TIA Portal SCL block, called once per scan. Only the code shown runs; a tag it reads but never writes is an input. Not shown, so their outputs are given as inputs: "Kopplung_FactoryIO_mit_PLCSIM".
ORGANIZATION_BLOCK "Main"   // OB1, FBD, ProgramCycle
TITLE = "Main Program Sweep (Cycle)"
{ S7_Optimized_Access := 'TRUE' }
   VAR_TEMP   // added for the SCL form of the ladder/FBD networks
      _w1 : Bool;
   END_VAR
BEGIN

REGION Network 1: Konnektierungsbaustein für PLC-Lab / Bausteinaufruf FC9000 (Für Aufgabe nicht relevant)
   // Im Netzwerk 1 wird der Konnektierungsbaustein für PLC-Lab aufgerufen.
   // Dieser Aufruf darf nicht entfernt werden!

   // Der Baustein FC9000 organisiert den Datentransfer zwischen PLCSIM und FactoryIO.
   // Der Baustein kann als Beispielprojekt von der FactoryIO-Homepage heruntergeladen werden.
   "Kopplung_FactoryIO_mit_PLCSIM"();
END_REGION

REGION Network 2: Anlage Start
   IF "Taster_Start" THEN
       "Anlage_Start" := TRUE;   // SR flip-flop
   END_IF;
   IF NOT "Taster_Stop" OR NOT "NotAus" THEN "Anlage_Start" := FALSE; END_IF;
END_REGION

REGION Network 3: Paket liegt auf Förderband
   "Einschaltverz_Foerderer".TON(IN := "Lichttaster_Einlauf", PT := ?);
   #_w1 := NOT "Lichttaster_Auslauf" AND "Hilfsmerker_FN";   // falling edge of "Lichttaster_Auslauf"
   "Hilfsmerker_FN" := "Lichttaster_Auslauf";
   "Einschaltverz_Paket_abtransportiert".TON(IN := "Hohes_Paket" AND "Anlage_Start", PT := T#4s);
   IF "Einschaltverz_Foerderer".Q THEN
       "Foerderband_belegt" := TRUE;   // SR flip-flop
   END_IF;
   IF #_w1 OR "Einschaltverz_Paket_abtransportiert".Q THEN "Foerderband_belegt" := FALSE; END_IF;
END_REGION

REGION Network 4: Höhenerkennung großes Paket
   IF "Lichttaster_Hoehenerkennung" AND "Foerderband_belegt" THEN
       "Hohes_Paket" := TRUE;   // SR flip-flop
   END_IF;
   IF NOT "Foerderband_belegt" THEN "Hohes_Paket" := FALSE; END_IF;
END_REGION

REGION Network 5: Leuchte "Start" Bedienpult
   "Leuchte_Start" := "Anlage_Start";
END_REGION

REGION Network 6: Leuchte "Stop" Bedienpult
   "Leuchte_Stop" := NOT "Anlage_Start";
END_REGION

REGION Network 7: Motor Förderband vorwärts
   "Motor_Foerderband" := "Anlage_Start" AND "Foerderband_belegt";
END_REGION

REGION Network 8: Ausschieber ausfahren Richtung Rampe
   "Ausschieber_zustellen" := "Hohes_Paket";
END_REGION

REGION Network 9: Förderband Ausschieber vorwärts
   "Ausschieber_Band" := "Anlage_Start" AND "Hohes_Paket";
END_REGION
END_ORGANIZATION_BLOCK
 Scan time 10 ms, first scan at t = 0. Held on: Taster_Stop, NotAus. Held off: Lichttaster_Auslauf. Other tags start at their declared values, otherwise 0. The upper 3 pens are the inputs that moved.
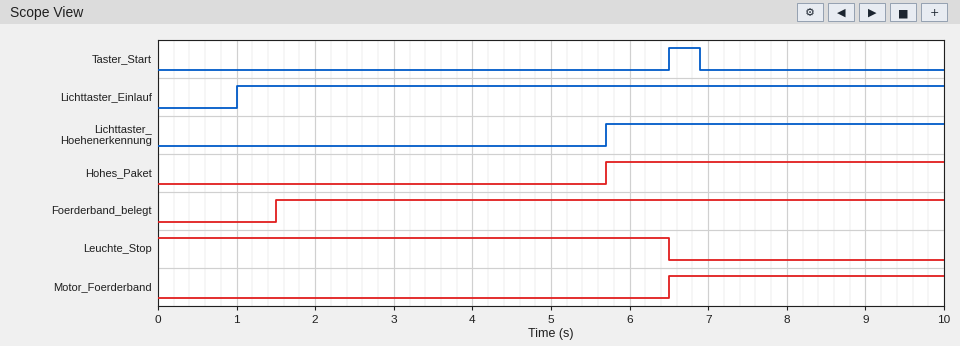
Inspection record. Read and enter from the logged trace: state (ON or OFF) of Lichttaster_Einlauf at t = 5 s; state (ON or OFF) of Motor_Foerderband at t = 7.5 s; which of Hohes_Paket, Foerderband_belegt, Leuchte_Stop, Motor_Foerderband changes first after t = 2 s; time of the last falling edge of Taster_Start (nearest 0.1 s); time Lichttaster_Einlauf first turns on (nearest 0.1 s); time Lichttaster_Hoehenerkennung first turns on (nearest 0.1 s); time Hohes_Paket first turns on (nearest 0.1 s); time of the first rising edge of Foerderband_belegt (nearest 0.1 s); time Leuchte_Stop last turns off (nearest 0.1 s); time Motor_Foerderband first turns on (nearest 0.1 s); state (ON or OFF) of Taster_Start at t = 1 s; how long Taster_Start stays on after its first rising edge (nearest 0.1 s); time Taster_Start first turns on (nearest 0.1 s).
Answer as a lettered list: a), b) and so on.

a) ON
b) ON
c) Hohes_Paket
d) 6.9 s
e) 1.0 s
f) 5.7 s
g) 5.7 s
h) 1.5 s
i) 6.5 s
j) 6.5 s
k) OFF
l) 0.4 s
m) 6.5 s
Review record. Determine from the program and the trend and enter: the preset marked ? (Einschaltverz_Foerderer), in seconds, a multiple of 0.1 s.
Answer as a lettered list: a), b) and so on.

a) 0.5 s
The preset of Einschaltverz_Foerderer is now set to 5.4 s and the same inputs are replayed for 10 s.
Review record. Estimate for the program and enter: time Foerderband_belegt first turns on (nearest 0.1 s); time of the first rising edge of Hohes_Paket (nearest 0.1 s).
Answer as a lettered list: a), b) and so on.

a) 6.4 s
b) 6.4 s
